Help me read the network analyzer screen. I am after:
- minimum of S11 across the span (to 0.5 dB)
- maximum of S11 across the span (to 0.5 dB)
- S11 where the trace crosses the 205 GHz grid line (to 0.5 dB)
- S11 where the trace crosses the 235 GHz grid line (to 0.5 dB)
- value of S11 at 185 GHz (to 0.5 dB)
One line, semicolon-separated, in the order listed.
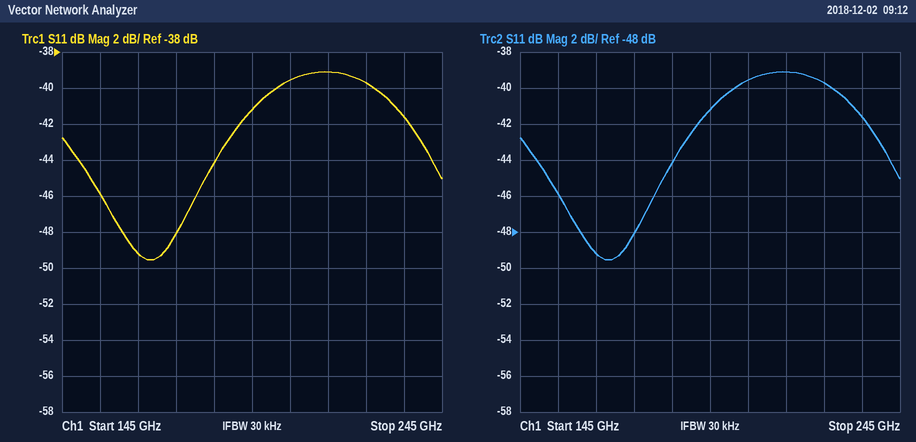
-49.5 dB; -39.0 dB; -39.5 dB; -41.5 dB; -44.0 dB
